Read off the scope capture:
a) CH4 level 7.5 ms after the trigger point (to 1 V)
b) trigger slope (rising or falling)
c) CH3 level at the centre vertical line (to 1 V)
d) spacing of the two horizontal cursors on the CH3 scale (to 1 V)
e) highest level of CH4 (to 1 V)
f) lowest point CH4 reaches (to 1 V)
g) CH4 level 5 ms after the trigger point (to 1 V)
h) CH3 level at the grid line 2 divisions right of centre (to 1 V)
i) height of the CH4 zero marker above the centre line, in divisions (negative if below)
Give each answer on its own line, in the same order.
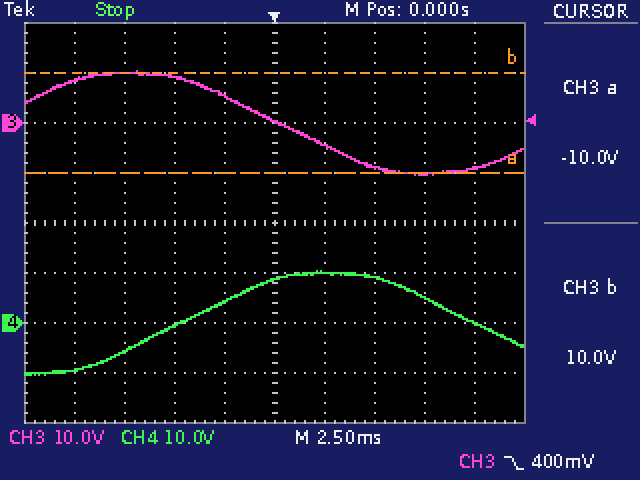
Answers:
5 V
falling
0 V
20 V
10 V
-10 V
9 V
-9 V
-2.0 div
